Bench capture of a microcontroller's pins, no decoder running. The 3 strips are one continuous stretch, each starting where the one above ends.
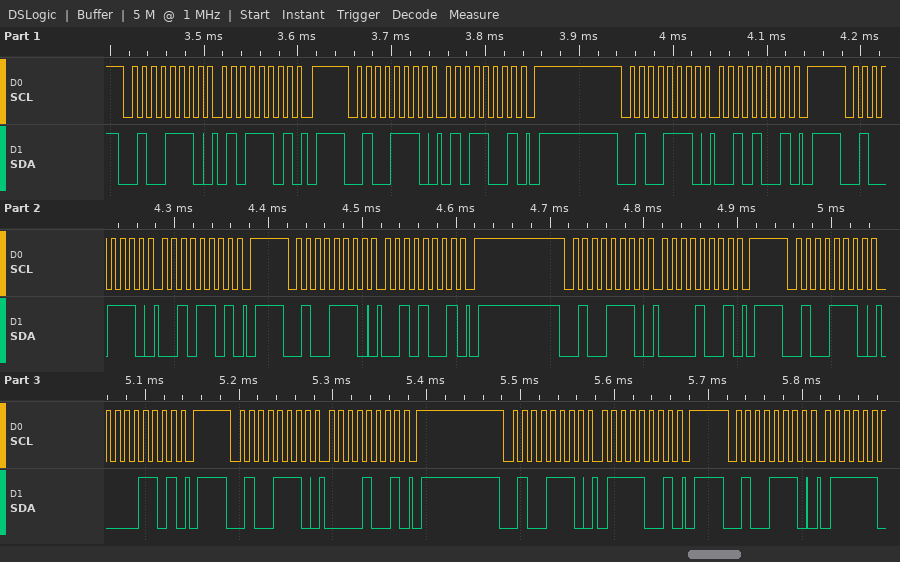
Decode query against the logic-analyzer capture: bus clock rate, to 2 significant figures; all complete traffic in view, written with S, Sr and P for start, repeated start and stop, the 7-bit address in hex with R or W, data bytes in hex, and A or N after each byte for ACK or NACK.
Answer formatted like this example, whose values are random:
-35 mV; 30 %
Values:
100 kHz; S 27W A 5D A P S 27W A 59 A P S 27W A 29 A P S 27W A 2D A P S 27W A 29 A P S 27W A 09 A P S 27W A 0D A P S 27W A 09 A P S 27W A 79 A P S 27W A
